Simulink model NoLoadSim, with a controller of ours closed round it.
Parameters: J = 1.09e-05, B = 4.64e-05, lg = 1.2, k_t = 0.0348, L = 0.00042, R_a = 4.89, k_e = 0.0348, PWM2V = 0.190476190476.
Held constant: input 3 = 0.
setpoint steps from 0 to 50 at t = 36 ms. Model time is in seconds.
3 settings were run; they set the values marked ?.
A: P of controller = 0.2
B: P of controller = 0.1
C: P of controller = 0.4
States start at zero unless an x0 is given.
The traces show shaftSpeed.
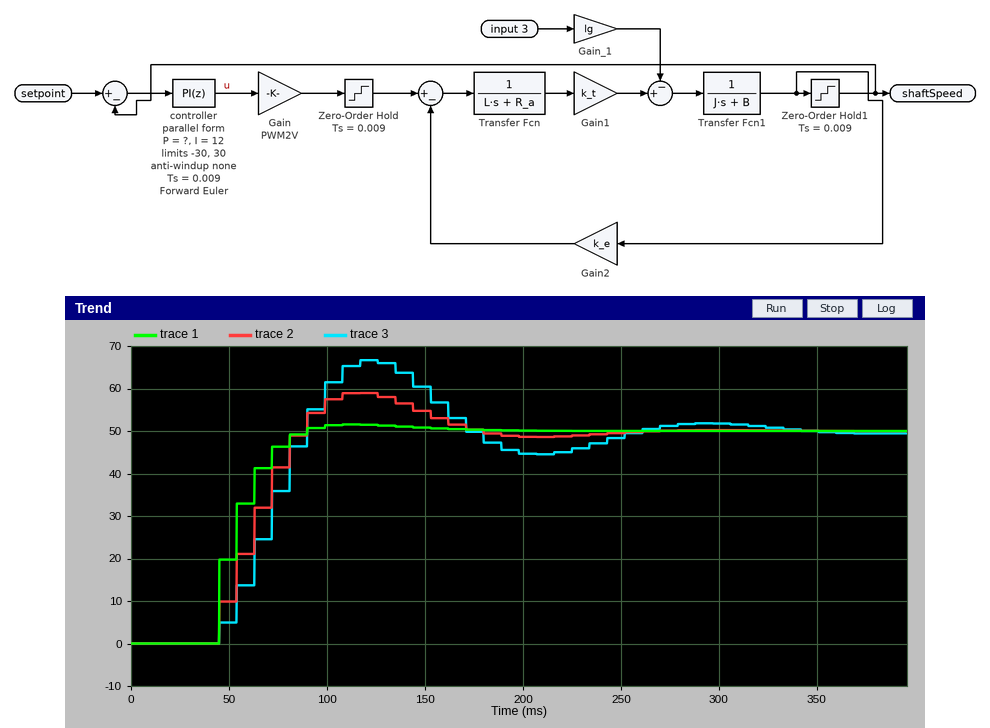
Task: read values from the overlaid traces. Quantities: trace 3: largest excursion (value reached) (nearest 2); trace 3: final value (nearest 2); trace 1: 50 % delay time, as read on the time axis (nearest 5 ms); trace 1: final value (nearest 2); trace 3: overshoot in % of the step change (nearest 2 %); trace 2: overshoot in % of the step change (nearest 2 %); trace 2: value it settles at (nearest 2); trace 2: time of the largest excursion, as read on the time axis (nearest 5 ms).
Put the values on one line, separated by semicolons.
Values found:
66; 50; 55 ms; 50; 34 %; 18 %; 50; 115 ms
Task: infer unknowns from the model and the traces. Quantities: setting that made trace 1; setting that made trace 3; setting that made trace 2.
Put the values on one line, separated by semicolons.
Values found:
C; B; A
